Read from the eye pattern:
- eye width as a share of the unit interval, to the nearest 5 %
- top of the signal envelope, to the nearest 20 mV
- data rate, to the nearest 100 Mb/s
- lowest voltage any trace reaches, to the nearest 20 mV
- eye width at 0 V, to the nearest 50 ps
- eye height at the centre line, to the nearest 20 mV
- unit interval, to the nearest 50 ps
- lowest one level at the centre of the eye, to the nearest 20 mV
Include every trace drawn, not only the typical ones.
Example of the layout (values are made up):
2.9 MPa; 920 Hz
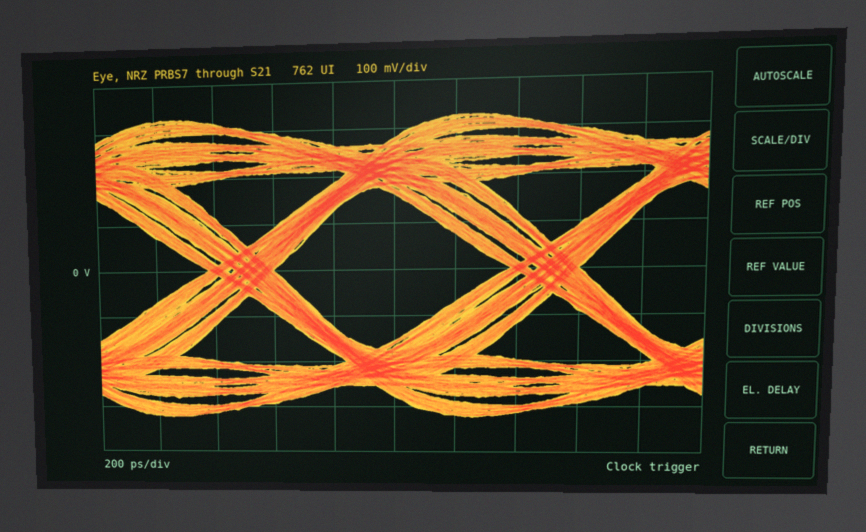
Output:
80 %; 320 mV; 1.0 Gb/s; -320 mV; 800 ps; 320 mV; 1.00 ns; 160 mV
